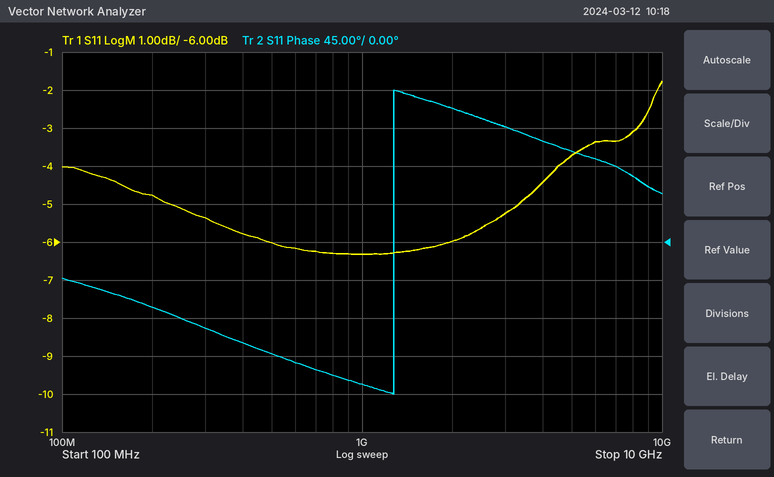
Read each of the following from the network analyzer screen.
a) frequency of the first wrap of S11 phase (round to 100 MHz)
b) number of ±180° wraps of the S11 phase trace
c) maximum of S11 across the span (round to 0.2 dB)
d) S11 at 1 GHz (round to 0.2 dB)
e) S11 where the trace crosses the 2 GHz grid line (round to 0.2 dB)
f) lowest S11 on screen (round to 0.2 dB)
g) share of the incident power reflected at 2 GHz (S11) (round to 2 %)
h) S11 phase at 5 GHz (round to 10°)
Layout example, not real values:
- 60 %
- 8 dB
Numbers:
- 1.3 GHz
- 1
- -1.8 dB
- -6.4 dB
- -6.0 dB
- -6.4 dB
- 26 %
- 110°
